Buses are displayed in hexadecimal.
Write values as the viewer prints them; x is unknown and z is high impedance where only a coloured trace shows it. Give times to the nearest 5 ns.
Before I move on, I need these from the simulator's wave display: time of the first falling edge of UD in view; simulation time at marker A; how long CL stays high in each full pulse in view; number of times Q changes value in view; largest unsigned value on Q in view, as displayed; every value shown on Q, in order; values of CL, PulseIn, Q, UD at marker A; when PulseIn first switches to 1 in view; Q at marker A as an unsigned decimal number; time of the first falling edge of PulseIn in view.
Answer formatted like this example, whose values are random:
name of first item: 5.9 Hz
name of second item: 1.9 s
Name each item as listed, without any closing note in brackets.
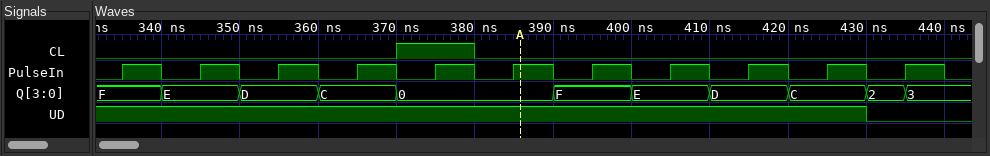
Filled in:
time of the first falling edge of UD in view: 430 ns
simulation time at marker A: 385 ns
how long CL stays high in each full pulse in view: 10 ns
number of times Q changes value in view: 10
largest unsigned value on Q in view, as displayed: F
every value shown on Q, in order: F, E, D, C, 0, F, E, D, C, 2, 3
values of CL, PulseIn, Q, UD at marker A: CL=0, PulseIn=1, Q=0, UD=1
when PulseIn first switches to 1 in view: 335 ns
Q at marker A as an unsigned decimal number: 0
time of the first falling edge of PulseIn in view: 340 ns
